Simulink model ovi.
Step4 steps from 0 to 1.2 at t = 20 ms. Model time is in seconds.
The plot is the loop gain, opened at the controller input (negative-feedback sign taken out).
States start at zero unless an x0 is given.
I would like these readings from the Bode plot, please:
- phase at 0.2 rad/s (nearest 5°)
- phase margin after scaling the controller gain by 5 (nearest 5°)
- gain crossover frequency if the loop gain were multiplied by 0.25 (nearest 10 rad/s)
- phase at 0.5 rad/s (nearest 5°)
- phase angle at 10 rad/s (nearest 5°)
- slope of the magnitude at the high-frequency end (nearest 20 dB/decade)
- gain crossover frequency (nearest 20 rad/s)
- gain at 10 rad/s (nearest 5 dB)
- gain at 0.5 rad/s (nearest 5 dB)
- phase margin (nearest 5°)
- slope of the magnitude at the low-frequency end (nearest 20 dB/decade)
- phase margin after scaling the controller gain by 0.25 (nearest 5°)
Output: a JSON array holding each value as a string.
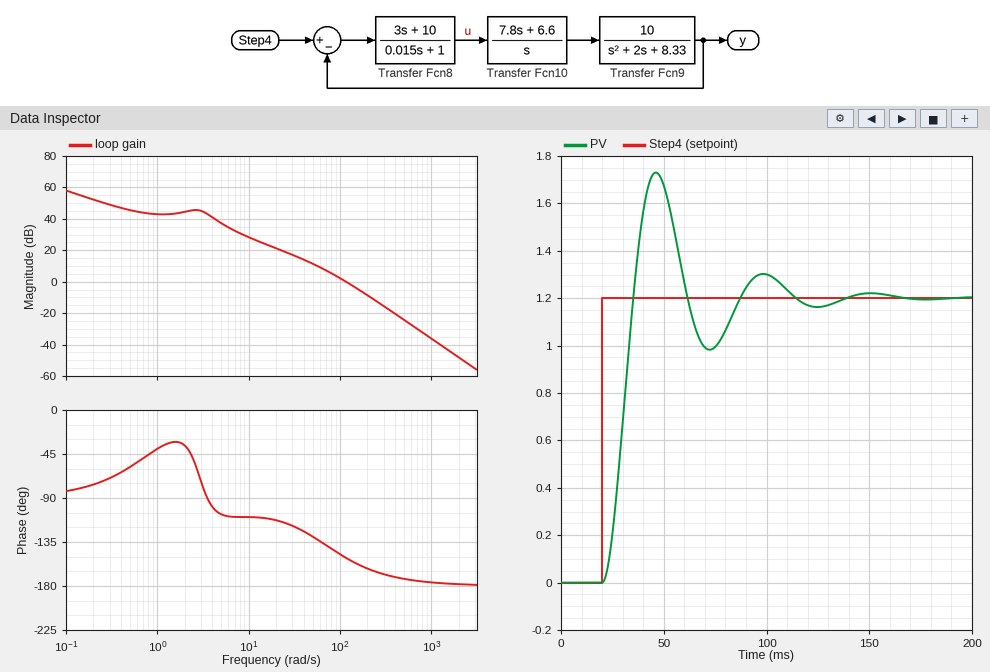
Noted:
["-75°", "15°", "50 rad/s", "-60°", "-110°", "-40 dB/decade", "120 rad/s", "30 dB", "45 dB", "30°", "-20 dB/decade", "50°"]
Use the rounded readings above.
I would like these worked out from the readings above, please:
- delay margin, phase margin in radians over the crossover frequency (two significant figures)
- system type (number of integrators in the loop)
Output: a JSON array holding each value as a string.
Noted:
["0.0044 s", "1"]
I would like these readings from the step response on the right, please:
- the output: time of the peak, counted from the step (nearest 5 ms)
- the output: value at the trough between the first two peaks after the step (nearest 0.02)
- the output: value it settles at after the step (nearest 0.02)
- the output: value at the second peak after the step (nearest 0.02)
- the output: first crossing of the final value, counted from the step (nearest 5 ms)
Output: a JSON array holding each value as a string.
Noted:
["25 ms", "0.98", "1.20", "1.30", "15 ms"]
